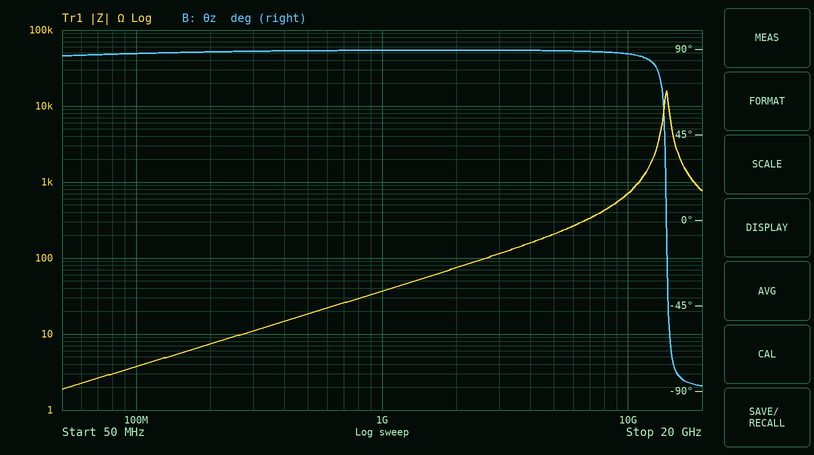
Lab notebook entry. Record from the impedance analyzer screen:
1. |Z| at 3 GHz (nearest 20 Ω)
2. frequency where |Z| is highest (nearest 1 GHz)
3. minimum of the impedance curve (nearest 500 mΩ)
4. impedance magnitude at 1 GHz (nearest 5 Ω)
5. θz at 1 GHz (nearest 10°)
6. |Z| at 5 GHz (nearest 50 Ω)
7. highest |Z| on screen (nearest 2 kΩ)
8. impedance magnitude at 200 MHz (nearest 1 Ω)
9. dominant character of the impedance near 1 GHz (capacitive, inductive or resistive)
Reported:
120 Ω
14 GHz
2.0 Ω
35 Ω
90°
200 Ω
16 kΩ
7 Ω
inductive
